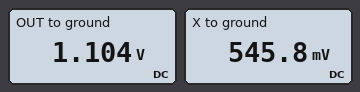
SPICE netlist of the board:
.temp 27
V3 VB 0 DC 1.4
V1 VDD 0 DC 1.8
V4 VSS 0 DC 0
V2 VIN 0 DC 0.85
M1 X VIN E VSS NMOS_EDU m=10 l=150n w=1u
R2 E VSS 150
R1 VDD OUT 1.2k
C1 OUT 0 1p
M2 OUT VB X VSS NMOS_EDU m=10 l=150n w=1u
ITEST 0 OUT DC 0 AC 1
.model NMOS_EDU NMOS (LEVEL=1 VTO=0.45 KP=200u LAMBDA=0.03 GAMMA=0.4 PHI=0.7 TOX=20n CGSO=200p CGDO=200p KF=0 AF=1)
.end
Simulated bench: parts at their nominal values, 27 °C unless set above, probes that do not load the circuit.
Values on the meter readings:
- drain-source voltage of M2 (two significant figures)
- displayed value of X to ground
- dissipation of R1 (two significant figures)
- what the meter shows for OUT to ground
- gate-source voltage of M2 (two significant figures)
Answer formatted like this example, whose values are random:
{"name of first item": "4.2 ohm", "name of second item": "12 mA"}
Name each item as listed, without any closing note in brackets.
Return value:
{"drain-source voltage of M2": "560 mV", "displayed value of X to ground": "545.8 mV", "dissipation of R1": "400 µW", "what the meter shows for OUT to ground": "1.104 V", "gate-source voltage of M2": "850 mV"}
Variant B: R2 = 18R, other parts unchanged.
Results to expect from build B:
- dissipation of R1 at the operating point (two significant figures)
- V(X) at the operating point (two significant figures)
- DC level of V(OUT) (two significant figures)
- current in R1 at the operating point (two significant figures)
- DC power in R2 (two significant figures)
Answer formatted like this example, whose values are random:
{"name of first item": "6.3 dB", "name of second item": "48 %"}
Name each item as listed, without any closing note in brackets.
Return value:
{"dissipation of R1 at the operating point": "1.1 mW", "V(X) at the operating point": "420 mV", "DC level of V(OUT)": "640 mV", "current in R1 at the operating point": "970 µA", "DC power in R2": "17 µW"}
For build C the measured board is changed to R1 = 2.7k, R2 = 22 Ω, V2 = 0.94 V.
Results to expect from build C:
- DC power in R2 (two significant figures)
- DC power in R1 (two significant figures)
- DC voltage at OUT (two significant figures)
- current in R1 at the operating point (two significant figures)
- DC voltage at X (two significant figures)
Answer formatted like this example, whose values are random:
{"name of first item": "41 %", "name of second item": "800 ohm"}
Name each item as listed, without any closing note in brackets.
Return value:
{"DC power in R2": "7.9 µW", "DC power in R1": "970 µW", "DC voltage at OUT": "180 mV", "current in R1 at the operating point": "600 µA", "DC voltage at X": "120 mV"}
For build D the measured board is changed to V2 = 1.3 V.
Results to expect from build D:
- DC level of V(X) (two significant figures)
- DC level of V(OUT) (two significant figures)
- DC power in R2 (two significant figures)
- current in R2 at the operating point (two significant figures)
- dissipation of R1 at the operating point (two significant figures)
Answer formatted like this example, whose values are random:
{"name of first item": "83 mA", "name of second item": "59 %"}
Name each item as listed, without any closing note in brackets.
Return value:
{"DC level of V(X)": "310 mV", "DC level of V(OUT)": "480 mV", "DC power in R2": "180 µW", "current in R2 at the operating point": "1.1 mA", "dissipation of R1 at the operating point": "1.5 mW"}
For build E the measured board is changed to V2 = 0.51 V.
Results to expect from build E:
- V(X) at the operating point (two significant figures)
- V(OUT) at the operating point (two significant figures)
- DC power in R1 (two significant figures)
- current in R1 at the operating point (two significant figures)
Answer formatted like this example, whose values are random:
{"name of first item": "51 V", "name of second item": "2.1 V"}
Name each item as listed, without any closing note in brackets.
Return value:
{"V(X) at the operating point": "750 mV", "V(OUT) at the operating point": "1.8 V", "DC power in R1": "550 nW", "current in R1 at the operating point": "21 µA"}
